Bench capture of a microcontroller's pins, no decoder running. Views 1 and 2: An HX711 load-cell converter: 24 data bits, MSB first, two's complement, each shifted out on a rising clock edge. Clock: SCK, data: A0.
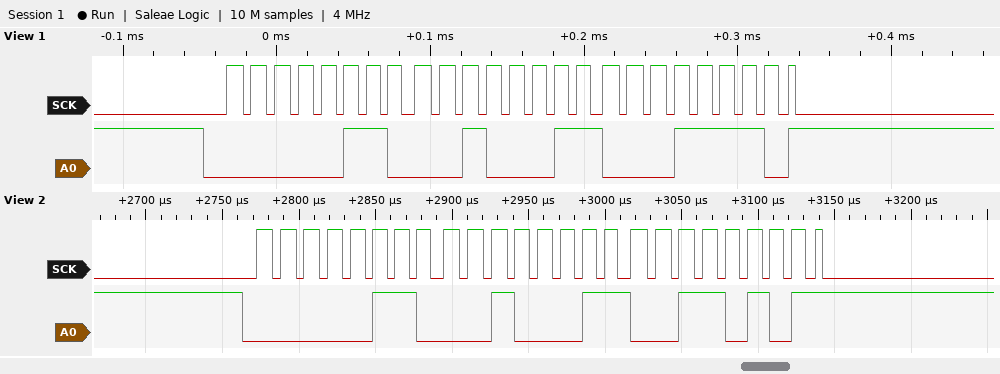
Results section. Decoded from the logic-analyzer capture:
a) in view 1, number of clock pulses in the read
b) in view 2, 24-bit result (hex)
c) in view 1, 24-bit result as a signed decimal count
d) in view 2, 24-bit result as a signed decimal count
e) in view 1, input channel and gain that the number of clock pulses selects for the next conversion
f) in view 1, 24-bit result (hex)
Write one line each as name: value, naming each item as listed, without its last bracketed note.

in view 1, number of clock pulses in the read: 25
in view 2, 24-bit result: 0x062335
in view 1, 24-bit result as a signed decimal count: 402206
in view 2, 24-bit result as a signed decimal count: 402229
in view 1, input channel and gain that the number of clock pulses selects for the next conversion: channel A, gain 128
in view 1, 24-bit result: 0x06231E
